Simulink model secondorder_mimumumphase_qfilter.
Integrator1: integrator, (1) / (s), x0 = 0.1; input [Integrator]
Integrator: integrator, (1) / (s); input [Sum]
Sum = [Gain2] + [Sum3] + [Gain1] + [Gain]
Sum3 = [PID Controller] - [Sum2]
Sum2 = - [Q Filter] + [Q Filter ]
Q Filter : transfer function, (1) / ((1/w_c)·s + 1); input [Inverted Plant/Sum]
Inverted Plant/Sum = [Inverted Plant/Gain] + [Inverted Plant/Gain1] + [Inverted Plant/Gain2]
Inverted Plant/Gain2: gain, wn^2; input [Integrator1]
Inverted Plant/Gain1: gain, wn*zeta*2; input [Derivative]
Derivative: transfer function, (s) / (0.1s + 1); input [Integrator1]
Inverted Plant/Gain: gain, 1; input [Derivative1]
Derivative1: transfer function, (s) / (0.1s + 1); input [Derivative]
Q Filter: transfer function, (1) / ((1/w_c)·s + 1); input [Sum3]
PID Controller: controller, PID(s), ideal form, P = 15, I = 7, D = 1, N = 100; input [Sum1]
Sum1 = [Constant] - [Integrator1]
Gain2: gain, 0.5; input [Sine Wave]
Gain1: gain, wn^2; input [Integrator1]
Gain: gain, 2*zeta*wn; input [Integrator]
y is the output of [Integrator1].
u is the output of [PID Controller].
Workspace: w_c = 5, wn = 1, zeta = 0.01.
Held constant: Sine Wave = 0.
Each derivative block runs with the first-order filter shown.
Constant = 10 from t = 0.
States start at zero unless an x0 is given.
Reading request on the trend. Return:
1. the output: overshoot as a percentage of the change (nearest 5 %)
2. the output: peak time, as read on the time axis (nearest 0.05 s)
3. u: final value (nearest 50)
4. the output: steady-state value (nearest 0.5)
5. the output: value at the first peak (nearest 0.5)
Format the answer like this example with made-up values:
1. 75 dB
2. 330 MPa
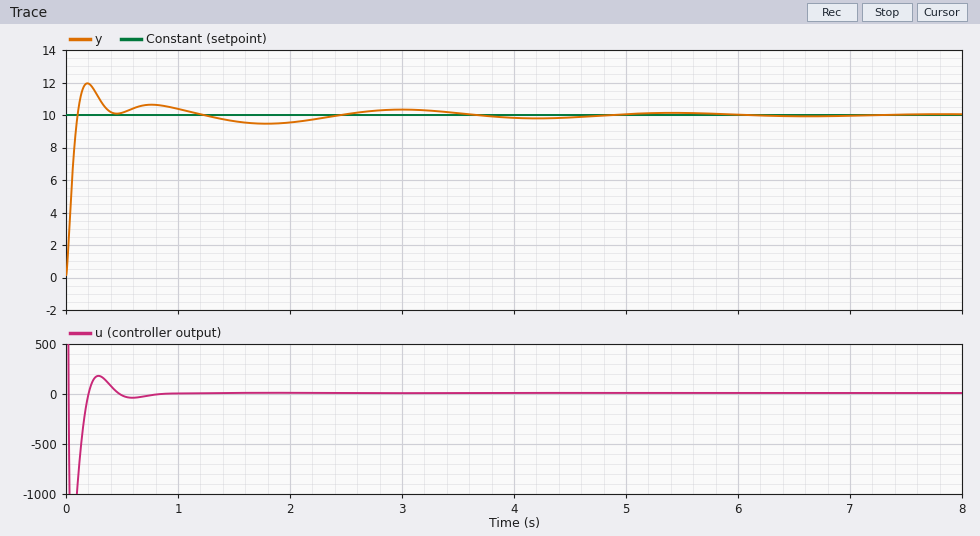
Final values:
1. 20 %
2. 0.20 s
3. 0
4. 10.0
5. 12.0
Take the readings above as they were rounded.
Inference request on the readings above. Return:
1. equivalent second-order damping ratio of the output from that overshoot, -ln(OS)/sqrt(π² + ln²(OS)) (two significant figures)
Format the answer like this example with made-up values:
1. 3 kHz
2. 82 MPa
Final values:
1. 0.46
